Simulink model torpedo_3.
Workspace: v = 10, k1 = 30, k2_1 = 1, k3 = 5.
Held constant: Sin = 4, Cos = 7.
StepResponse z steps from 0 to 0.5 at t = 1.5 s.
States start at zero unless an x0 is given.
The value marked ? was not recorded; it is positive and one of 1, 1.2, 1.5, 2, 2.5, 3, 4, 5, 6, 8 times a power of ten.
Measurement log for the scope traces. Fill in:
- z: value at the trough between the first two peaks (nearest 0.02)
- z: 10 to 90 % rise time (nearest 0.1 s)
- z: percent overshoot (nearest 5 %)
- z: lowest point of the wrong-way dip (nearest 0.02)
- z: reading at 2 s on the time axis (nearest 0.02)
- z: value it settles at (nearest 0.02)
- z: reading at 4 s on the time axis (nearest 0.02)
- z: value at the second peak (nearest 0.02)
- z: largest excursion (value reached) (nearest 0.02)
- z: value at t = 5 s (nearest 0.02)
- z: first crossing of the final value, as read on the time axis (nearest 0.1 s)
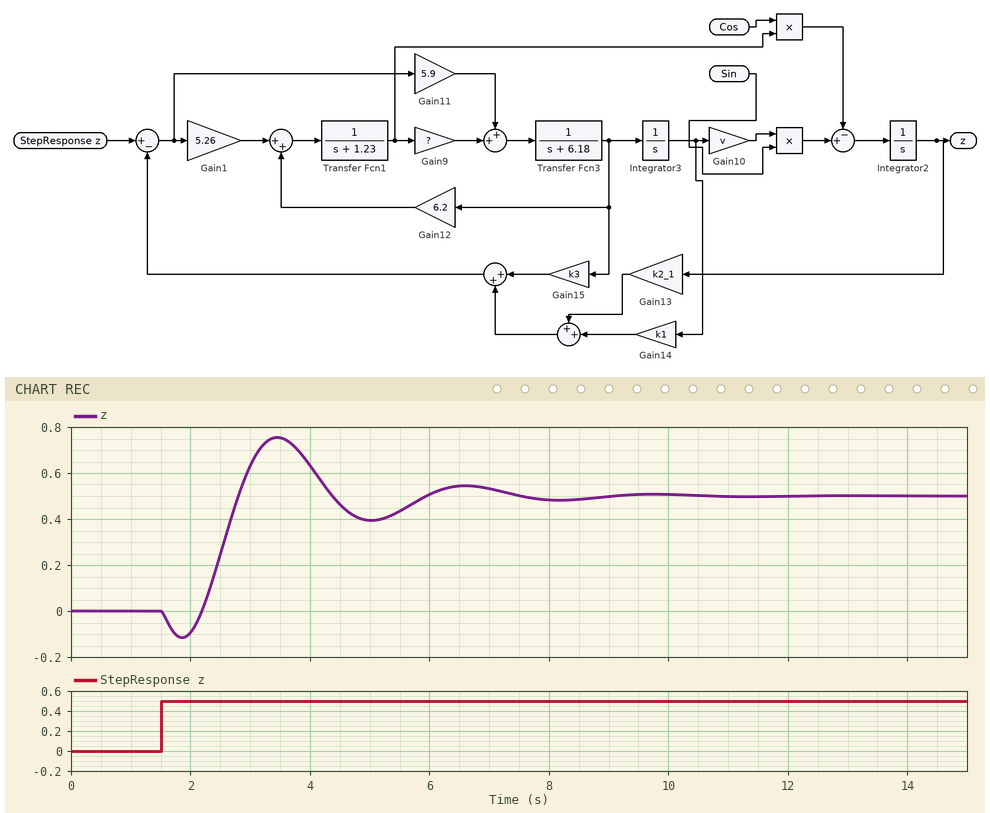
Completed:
0.40
0.5 s
50 %
-0.12
-0.10
0.50
0.64
0.54
0.76
0.40
2.8 s
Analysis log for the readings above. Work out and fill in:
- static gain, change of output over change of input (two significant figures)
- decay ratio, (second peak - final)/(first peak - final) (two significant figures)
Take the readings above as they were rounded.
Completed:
1.0
0.15
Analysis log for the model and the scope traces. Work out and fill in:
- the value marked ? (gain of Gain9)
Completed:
2.5
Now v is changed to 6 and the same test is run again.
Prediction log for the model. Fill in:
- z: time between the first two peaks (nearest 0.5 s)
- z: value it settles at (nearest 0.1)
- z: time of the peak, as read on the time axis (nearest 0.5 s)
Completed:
4.0 s
0.5
4.0 s
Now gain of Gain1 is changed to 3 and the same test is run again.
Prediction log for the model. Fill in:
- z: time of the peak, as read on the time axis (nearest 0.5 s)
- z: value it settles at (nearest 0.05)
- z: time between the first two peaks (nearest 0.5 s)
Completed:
3.5 s
0.50
3.5 s
